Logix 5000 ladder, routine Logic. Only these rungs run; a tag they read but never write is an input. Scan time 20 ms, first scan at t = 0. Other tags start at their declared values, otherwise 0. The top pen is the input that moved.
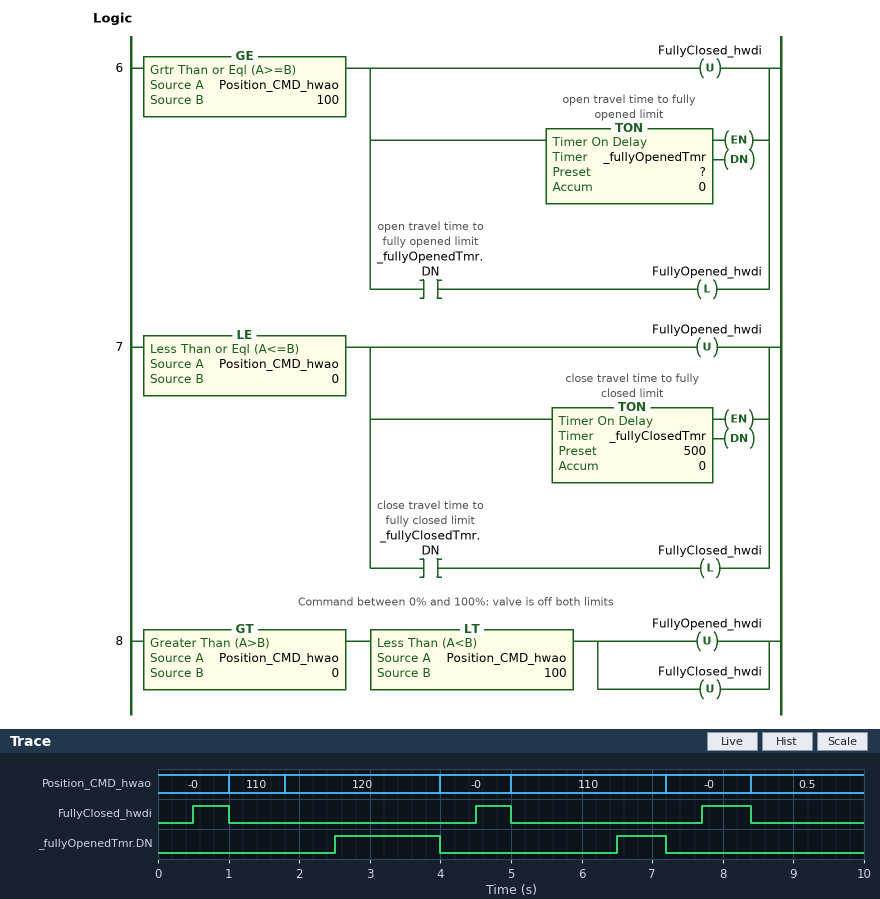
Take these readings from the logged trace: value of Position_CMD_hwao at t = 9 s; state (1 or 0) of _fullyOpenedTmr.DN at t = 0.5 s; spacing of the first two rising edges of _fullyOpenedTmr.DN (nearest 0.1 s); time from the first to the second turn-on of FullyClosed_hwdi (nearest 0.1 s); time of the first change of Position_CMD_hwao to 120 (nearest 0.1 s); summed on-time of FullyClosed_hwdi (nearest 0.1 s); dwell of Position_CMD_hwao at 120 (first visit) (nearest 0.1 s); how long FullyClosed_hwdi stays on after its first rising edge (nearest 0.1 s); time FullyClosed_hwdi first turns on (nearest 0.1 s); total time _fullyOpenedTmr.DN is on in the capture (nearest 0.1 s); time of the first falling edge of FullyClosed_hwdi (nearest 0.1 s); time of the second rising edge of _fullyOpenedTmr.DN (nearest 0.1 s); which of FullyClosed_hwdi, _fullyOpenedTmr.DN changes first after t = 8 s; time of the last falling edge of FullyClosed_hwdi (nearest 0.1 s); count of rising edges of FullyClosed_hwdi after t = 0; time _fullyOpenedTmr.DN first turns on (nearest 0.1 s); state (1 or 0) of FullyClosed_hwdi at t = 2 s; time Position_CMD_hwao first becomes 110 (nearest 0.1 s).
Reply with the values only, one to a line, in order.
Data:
0.5
0
4.0 s
4.0 s
1.8 s
1.7 s
2.2 s
0.5 s
0.5 s
2.2 s
1.0 s
6.5 s
FullyClosed_hwdi
8.4 s
3
2.5 s
0
1.0 s
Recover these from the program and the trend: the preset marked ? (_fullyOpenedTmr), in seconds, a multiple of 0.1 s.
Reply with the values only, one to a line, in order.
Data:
1.5 s
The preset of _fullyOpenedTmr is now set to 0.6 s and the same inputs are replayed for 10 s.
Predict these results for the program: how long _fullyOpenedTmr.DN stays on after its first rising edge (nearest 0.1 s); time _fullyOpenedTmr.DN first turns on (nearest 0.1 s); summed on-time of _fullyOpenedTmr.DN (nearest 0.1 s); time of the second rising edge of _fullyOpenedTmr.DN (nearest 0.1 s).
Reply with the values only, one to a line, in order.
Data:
2.4 s
1.6 s
4.0 s
5.6 s
